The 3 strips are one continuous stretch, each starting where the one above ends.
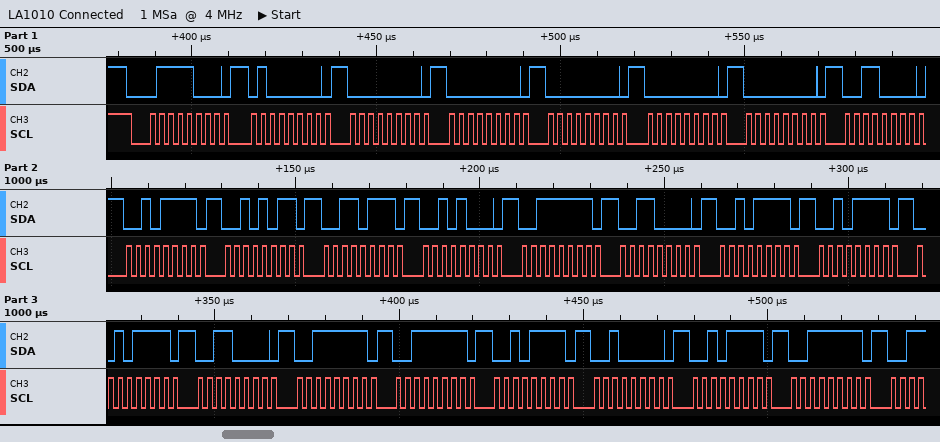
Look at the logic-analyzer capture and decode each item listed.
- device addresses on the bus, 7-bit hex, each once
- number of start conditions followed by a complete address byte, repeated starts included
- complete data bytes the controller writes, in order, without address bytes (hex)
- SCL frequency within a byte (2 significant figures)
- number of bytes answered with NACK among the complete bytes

0x3C
1
40 00 00 00 00 00 30 2F 2B 37 28 3F 30 2F 2F 2F 30 3F 3F 2F 20 2F 3F
400 kHz
0
